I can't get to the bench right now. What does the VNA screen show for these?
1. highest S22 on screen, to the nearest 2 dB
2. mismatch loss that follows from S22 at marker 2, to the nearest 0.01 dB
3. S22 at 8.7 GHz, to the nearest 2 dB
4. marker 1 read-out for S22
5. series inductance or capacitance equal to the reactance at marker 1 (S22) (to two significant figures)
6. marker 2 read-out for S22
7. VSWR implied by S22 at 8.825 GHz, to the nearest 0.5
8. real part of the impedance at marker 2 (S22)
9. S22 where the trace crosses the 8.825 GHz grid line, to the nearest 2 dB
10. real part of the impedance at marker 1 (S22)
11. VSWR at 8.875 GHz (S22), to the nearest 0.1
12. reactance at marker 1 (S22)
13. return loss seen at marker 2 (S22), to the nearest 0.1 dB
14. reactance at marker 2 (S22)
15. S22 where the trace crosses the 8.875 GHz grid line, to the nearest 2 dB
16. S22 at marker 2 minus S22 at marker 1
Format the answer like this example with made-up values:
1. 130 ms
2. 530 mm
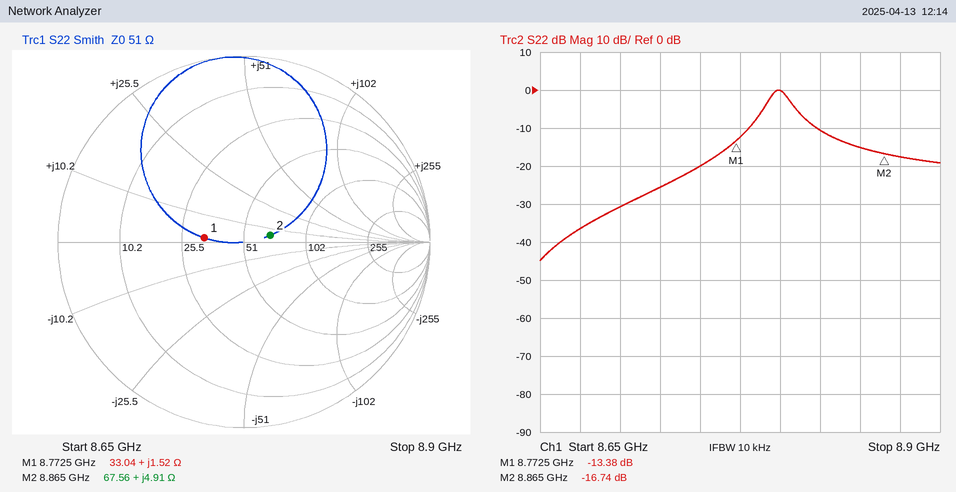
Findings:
1. 0 dB
2. 0.09 dB
3. -30 dB
4. -13.38 dB
5. 28 pH
6. -16.74 dB
7. 2.0
8. 67.56 Ω
9. -10 dB
10. 33.04 Ω
11. 1.3
12. +1.52 Ω
13. 16.7 dB
14. +4.91 Ω
15. -18 dB
16. -3.36 dB
